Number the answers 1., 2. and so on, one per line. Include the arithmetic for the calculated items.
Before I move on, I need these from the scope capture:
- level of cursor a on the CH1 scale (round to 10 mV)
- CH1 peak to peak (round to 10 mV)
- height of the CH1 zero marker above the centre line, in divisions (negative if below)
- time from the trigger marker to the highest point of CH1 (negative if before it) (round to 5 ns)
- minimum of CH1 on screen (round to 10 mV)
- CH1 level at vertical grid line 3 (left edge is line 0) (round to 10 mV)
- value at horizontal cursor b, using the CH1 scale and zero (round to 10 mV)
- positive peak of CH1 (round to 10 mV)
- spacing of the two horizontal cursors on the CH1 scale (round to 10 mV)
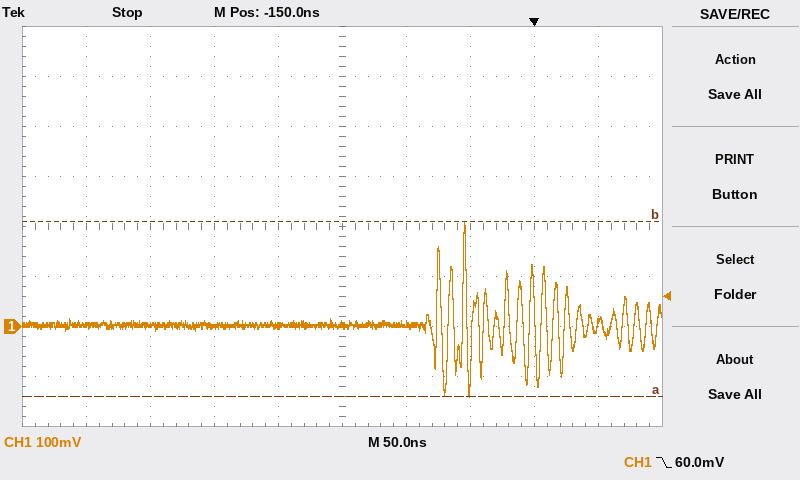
1. -140 mV
2. 210 mV − (-140 mV) = 350 mV
3. -2.0 div
4. -55 ns
5. -140 mV
6. 0 mV
7. 210 mV
8. 210 mV
9. 350 mV
